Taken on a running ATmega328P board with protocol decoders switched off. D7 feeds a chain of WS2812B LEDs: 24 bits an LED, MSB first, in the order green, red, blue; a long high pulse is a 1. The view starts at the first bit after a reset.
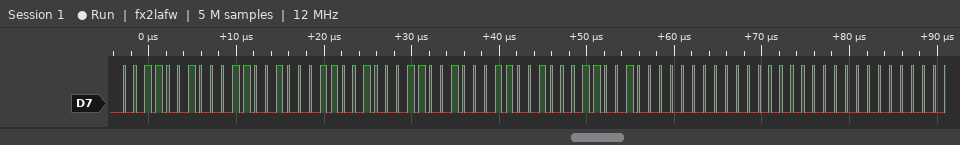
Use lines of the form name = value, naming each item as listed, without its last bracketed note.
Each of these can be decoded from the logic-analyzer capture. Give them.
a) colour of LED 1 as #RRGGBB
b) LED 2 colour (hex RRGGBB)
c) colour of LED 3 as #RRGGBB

colour of LED 1 as #RRGGBB = #323232
LED 2 colour = #323232
colour of LED 3 as #RRGGBB = #000000
